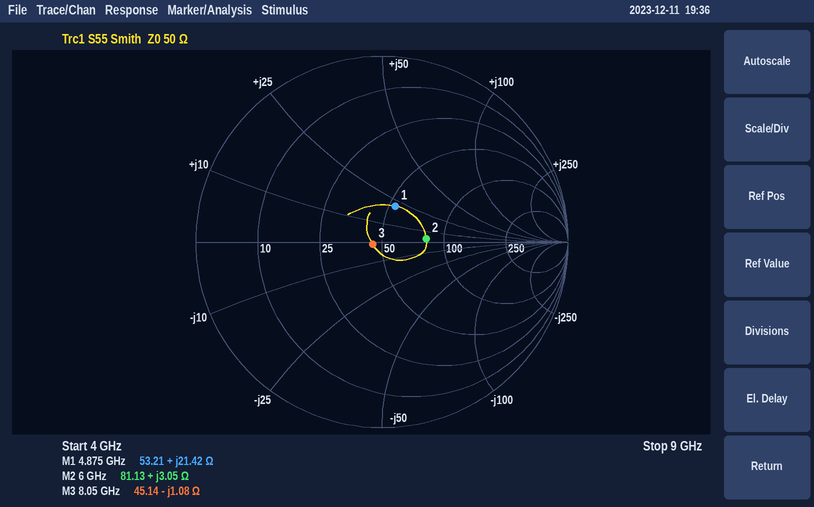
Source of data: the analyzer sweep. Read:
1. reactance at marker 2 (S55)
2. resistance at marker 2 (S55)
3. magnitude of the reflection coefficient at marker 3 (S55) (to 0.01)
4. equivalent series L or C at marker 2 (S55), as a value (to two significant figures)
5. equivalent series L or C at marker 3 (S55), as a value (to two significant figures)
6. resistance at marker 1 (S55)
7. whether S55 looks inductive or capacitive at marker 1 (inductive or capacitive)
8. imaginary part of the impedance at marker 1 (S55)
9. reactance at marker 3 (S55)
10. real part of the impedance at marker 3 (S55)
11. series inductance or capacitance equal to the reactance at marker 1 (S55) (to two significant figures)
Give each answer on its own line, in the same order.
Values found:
+3.05 Ω
81.13 Ω
0.05
81 pH
18 pF
53.21 Ω
inductive
+21.42 Ω
-1.08 Ω
45.14 Ω
700 pH
